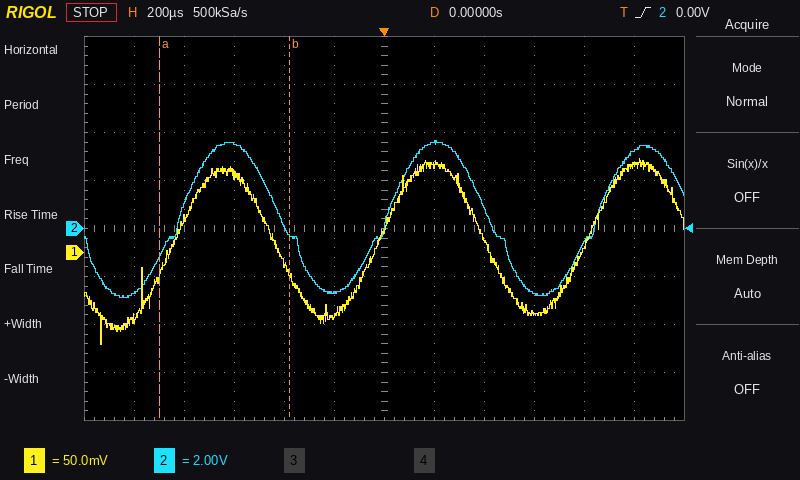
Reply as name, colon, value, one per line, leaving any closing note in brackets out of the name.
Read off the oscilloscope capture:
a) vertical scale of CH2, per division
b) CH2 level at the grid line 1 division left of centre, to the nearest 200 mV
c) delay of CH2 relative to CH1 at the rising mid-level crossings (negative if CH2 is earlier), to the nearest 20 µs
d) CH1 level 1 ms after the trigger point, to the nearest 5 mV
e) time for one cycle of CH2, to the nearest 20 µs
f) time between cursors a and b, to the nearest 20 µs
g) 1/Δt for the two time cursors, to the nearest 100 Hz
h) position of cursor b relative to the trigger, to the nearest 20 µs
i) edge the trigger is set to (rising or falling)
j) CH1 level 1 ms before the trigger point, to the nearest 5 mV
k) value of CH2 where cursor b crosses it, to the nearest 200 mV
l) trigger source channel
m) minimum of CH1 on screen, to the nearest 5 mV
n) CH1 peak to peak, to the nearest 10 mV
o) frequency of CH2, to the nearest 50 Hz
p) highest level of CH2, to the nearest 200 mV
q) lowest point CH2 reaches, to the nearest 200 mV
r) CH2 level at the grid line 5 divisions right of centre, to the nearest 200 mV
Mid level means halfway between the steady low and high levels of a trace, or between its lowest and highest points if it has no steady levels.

vertical scale of CH2, per division: 2 V
CH2 level at the grid line 1 division left of centre, to the nearest 200 mV: -2.6 V
delay of CH2 relative to CH1 at the rising mid-level crossings (negative if CH2 is earlier), to the nearest 20 µs: +40 µs
CH1 level 1 ms after the trigger point, to the nearest 5 mV: 90 mV
time for one cycle of CH2, to the nearest 20 µs: 840 µs
time between cursors a and b, to the nearest 20 µs: 520 µs
1/Δt for the two time cursors, to the nearest 100 Hz: 1.9 kHz
position of cursor b relative to the trigger, to the nearest 20 µs: -380 µs
edge the trigger is set to: rising
CH1 level 1 ms before the trigger point, to the nearest 5 mV: -70 mV
value of CH2 where cursor b crosses it, to the nearest 200 mV: -200 mV
trigger source channel: CH2
minimum of CH1 on screen, to the nearest 5 mV: -95 mV
CH1 peak to peak, to the nearest 10 mV: 190 mV
frequency of CH2, to the nearest 50 Hz: 1.20 kHz
highest level of CH2, to the nearest 200 mV: 3.6 V
lowest point CH2 reaches, to the nearest 200 mV: -2.8 V
CH2 level at the grid line 5 divisions right of centre, to the nearest 200 mV: 3.2 V
